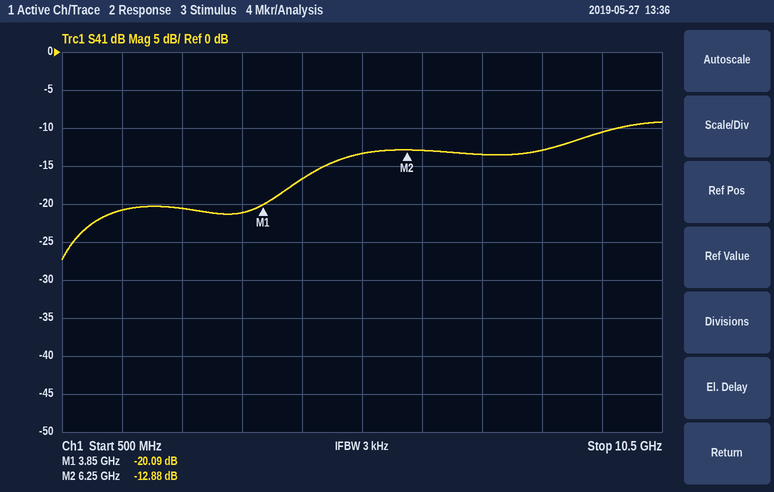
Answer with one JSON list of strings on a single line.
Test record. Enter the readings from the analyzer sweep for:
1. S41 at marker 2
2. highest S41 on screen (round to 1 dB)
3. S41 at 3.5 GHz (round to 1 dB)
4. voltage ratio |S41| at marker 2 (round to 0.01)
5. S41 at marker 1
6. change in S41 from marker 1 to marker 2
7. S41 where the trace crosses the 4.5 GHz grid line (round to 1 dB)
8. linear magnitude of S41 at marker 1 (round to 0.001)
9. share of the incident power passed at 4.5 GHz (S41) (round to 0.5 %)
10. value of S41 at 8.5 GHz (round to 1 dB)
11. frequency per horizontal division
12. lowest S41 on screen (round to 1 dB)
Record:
["-12.88 dB", "-9 dB", "-21 dB", "0.23", "-20.09 dB", "7.21 dB", "-17 dB", "0.099", "2.0 %", "-13 dB", "1 GHz", "-27 dB"]
